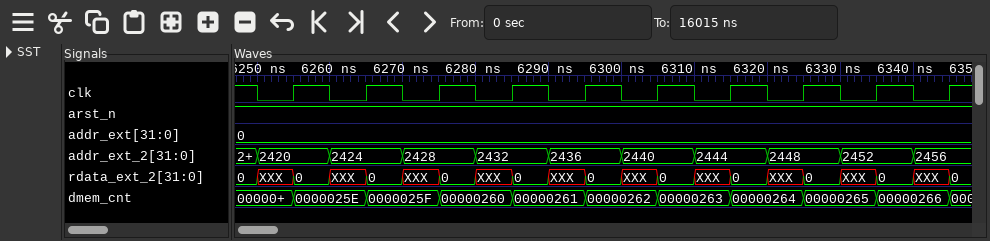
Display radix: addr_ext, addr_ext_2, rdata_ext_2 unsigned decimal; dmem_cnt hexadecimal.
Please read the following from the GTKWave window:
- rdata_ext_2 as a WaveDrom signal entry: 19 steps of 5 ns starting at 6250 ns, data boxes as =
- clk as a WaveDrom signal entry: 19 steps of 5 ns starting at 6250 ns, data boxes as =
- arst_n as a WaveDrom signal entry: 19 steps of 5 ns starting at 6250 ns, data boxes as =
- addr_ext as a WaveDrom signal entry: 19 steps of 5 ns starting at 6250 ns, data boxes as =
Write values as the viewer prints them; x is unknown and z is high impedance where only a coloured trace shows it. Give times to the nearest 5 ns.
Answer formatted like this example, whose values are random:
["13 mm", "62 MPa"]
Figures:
["{name: 'rdata_ext_2', wave: 'x=x=x=x=x=x=x=x=x=x', data: '0 0 0 0 0 0 0 0 0'}", "{name: 'clk', wave: '0101010101010101010'}", "{name: 'arst_n', wave: '1..................'}", "{name: 'addr_ext', wave: '=..................', data: '0'}"]
